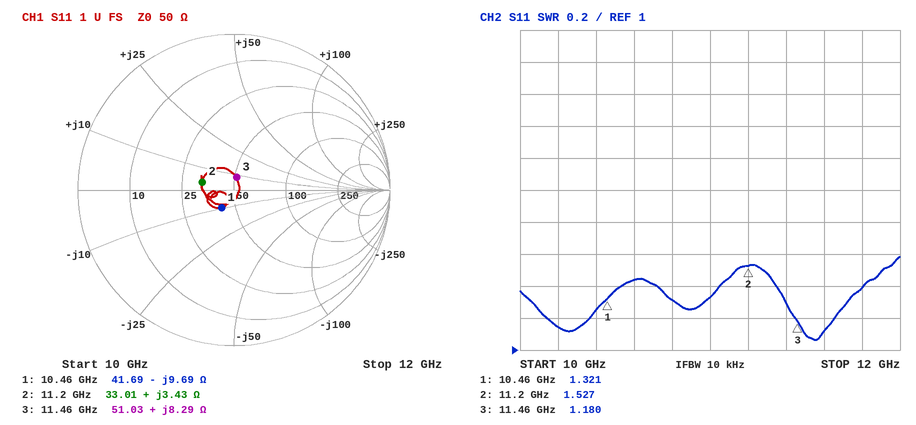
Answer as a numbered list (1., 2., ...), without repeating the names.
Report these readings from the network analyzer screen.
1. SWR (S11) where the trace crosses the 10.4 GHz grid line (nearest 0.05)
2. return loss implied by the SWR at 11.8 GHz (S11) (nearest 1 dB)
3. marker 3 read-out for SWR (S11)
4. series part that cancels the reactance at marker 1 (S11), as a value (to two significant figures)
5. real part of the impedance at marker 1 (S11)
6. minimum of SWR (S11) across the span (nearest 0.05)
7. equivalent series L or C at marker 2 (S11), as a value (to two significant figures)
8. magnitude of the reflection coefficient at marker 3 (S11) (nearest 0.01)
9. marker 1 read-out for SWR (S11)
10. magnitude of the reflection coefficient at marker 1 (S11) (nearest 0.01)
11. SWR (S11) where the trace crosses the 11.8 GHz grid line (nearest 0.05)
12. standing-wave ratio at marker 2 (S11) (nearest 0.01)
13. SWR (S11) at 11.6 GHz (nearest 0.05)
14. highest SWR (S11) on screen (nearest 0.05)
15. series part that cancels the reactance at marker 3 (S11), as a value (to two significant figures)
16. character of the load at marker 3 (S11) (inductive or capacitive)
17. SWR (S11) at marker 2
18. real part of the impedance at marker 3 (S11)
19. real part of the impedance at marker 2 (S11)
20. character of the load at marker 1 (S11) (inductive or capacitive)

1. 1.25
2. 16 dB
3. 1.180
4. 150 pH
5. 41.69 Ω
6. 1.05
7. 49 pH
8. 0.08
9. 1.321
10. 0.14
11. 1.40
12. 1.53
13. 1.10
14. 1.60
15. 1.7 pF
16. inductive
17. 1.527
18. 51.03 Ω
19. 33.01 Ω
20. capacitive
